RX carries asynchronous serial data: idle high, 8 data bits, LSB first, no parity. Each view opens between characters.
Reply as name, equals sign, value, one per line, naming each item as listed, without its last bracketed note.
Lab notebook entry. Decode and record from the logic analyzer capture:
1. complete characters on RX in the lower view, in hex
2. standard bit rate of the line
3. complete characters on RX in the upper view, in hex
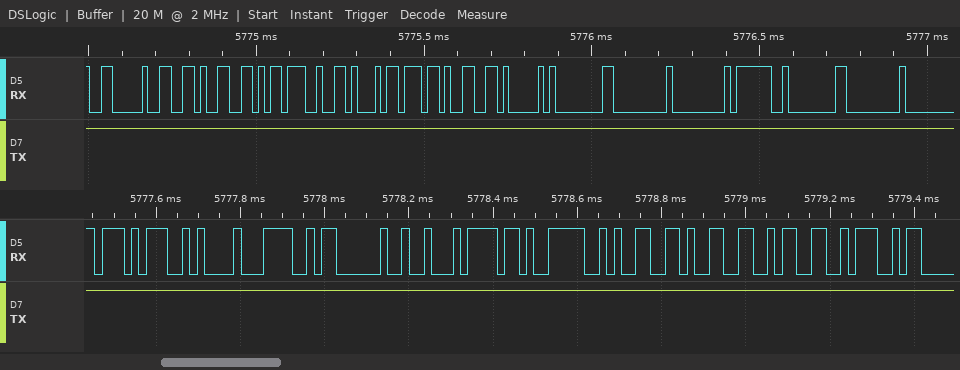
complete characters on RX in the lower view, in hex = D7, 0A, 3C, 03, 12, 6F, 3E, 99, 99, 9A, 3A
standard bit rate of the line = 57600 baud
complete characters on RX in the upper view, in hex = 06, 66, 66, 3B, 16, BB, 99, 41, 80, 00, 00, 3F, 80, 00
